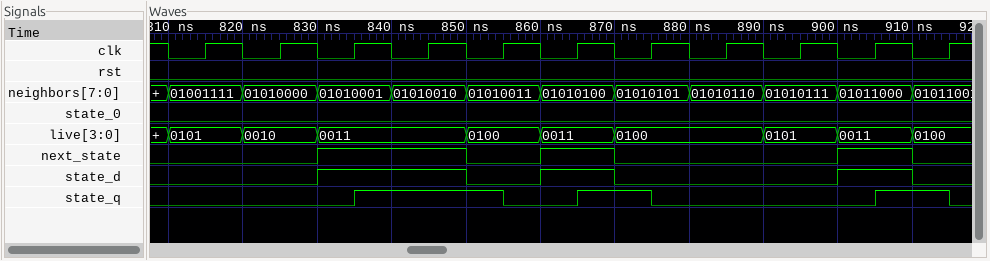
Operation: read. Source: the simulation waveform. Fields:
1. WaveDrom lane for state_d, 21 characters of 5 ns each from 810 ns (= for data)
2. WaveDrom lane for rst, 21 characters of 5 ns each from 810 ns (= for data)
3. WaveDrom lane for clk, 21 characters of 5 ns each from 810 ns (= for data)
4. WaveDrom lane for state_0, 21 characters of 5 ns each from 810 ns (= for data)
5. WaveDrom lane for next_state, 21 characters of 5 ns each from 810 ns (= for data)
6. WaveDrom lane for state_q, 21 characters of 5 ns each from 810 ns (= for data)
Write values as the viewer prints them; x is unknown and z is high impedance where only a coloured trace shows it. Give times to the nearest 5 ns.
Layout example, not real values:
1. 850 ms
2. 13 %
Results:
1. {name: 'state_d', wave: '0...1...0.1.0.....1.0'}
2. {name: 'rst', wave: '0....................'}
3. {name: 'clk', wave: '010101010101010101010'}
4. {name: 'state_0', wave: '0....................'}
5. {name: 'next_state', wave: '0...1...0.1.0.....1.0'}
6. {name: 'state_q', wave: '0....1...0.1.0.....1.'}
